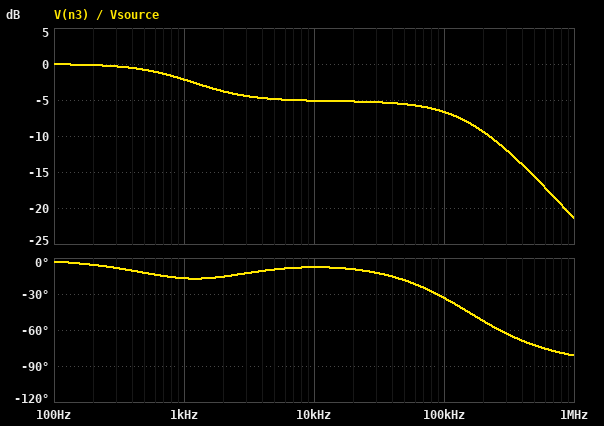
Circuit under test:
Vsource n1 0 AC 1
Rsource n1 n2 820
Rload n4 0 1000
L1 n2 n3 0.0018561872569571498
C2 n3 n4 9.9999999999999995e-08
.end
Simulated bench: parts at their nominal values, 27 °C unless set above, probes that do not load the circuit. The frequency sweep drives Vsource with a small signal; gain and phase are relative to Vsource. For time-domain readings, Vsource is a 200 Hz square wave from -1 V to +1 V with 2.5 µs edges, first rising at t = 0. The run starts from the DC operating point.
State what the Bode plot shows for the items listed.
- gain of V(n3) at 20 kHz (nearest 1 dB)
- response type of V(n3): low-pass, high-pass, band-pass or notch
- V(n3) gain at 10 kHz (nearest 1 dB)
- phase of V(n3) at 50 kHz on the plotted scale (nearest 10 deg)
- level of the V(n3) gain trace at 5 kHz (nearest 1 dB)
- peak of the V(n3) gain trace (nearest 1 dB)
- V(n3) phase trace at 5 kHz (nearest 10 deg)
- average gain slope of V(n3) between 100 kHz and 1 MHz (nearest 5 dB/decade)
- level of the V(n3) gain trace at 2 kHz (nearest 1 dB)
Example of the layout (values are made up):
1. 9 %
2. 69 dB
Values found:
1. -5 dB
2. low-pass
3. -5 dB
4. -20 deg
5. -5 dB
6. 0 dB
7. -10 deg
8. -15 dB/decade
9. -4 dB
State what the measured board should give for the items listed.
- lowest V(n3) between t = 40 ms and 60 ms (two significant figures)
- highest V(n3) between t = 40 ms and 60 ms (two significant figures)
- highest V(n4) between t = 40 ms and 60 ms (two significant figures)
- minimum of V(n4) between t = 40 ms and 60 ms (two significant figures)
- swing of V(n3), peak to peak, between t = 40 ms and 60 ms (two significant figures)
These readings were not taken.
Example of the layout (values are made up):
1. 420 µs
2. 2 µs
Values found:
1. -1.0 V
2. 1.0 V
3. 1.1 V
4. -1.1 V
5. 2.0 V
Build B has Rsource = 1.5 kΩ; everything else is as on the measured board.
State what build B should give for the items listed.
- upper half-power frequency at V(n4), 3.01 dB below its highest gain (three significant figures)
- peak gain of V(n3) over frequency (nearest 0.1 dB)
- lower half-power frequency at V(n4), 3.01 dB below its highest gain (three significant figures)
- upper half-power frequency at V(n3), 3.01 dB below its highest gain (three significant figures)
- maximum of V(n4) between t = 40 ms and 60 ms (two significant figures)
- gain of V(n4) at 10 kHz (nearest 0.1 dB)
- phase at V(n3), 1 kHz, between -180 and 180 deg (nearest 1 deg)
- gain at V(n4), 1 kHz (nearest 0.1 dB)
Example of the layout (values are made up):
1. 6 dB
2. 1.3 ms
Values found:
1. 215 kHz
2. 0 dB
3. 635 Hz
4. 775 Hz
5. 790 mV
6. -8.0 dB
7. -26 deg
8. -9.4 dB
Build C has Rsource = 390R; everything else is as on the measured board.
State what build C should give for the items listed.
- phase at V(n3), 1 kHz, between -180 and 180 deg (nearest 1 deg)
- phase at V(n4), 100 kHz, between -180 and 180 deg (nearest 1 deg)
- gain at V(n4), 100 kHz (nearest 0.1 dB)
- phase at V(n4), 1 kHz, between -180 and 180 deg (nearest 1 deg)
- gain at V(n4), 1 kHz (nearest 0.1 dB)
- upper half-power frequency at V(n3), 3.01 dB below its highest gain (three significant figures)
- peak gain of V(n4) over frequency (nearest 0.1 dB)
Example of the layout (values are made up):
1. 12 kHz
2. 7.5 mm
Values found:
1. -9 deg
2. -40 deg
3. -5.1 dB
4. 49 deg
5. -6.5 dB
6. 28.2 kHz
7. -2.9 dB
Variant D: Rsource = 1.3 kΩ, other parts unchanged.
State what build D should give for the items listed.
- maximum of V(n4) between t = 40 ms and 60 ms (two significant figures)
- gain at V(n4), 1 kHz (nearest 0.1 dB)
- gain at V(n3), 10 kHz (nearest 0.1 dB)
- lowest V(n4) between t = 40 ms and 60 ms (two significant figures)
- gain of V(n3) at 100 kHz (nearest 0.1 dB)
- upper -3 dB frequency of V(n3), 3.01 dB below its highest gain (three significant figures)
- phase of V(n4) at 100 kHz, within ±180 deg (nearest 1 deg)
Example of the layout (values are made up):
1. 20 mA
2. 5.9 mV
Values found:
1. 860 mV
2. -8.9 dB
3. -7.1 dB
4. -860 mV
5. -8.2 dB
6. 882 Hz
7. -27 deg
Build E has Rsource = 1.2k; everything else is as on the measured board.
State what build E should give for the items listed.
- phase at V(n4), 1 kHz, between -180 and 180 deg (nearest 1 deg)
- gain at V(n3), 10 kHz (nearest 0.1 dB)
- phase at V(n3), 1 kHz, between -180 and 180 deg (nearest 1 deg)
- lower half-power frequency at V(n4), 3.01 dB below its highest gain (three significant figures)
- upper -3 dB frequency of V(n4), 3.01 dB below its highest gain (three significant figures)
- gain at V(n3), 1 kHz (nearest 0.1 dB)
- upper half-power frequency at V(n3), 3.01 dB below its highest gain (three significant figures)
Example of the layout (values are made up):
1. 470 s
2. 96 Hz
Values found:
1. 36 deg
2. -6.7 dB
3. -22 deg
4. 721 Hz
5. 189 kHz
6. -3.2 dB
7. 951 Hz
